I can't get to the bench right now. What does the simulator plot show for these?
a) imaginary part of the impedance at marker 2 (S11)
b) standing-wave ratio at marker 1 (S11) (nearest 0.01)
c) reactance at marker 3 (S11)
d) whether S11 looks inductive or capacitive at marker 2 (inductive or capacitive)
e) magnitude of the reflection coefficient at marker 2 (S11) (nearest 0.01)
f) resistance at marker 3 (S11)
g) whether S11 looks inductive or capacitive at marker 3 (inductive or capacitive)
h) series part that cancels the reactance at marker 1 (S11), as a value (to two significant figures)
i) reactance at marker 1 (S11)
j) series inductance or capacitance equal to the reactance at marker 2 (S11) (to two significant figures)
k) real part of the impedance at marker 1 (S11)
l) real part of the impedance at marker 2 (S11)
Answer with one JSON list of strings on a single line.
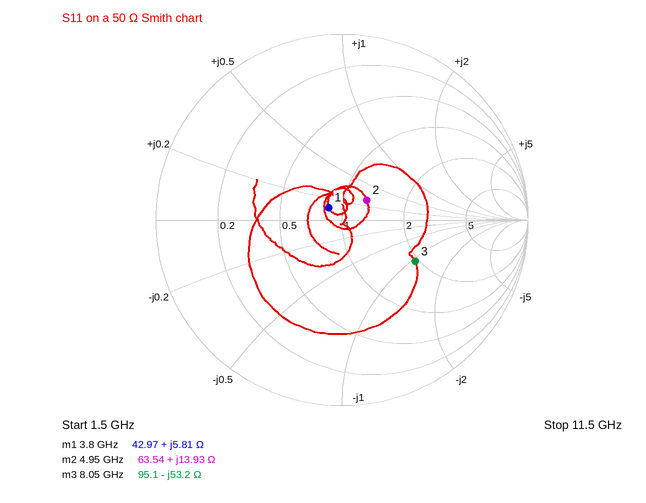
["+13.93 Ω", "1.22", "-53.2 Ω", "inductive", "0.17", "95.1 Ω", "capacitive", "7.2 pF", "+5.81 Ω", "450 pH", "42.97 Ω", "63.54 Ω"]
